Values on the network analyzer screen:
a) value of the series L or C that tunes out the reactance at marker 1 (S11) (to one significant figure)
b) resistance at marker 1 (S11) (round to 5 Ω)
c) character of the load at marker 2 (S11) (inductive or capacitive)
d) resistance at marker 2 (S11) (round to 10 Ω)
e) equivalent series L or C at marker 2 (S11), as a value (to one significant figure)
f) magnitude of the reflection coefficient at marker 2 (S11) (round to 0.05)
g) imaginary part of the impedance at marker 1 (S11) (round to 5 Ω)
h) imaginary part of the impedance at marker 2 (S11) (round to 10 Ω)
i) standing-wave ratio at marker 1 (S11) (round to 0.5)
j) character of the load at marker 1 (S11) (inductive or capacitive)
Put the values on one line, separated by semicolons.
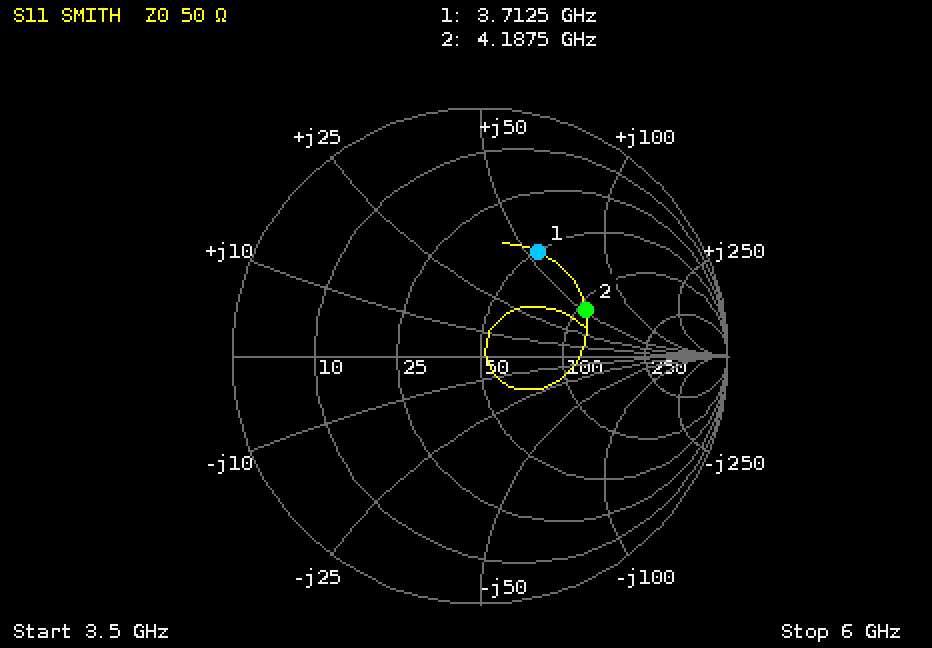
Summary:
800 fF; 50 Ω; inductive; 110 Ω; 2 nH; 0.45; +55 Ω; +50 Ω; 3.0; inductive
